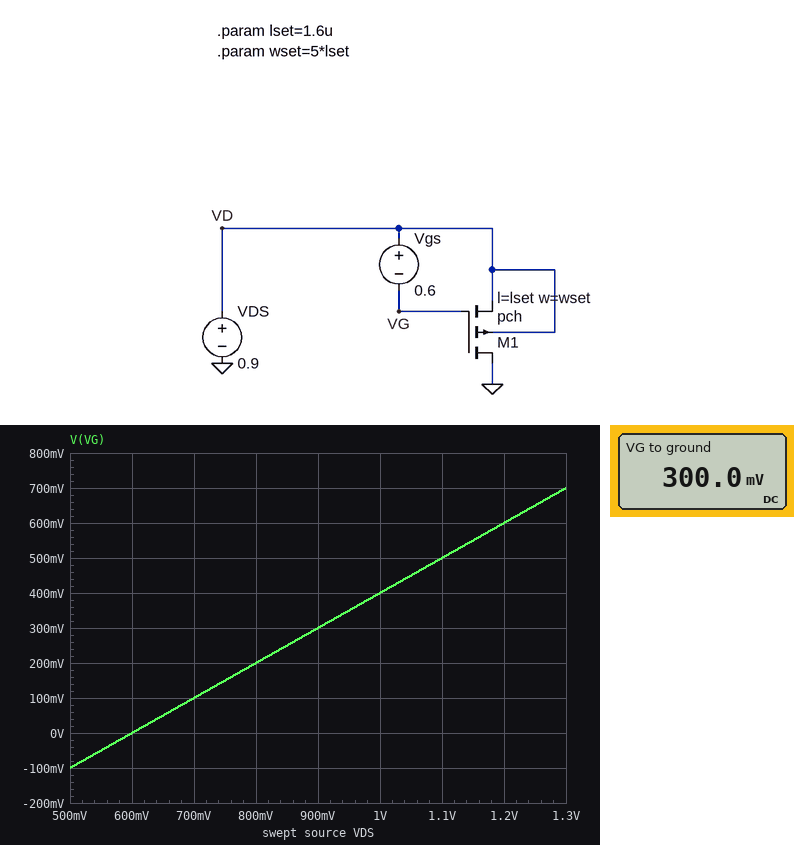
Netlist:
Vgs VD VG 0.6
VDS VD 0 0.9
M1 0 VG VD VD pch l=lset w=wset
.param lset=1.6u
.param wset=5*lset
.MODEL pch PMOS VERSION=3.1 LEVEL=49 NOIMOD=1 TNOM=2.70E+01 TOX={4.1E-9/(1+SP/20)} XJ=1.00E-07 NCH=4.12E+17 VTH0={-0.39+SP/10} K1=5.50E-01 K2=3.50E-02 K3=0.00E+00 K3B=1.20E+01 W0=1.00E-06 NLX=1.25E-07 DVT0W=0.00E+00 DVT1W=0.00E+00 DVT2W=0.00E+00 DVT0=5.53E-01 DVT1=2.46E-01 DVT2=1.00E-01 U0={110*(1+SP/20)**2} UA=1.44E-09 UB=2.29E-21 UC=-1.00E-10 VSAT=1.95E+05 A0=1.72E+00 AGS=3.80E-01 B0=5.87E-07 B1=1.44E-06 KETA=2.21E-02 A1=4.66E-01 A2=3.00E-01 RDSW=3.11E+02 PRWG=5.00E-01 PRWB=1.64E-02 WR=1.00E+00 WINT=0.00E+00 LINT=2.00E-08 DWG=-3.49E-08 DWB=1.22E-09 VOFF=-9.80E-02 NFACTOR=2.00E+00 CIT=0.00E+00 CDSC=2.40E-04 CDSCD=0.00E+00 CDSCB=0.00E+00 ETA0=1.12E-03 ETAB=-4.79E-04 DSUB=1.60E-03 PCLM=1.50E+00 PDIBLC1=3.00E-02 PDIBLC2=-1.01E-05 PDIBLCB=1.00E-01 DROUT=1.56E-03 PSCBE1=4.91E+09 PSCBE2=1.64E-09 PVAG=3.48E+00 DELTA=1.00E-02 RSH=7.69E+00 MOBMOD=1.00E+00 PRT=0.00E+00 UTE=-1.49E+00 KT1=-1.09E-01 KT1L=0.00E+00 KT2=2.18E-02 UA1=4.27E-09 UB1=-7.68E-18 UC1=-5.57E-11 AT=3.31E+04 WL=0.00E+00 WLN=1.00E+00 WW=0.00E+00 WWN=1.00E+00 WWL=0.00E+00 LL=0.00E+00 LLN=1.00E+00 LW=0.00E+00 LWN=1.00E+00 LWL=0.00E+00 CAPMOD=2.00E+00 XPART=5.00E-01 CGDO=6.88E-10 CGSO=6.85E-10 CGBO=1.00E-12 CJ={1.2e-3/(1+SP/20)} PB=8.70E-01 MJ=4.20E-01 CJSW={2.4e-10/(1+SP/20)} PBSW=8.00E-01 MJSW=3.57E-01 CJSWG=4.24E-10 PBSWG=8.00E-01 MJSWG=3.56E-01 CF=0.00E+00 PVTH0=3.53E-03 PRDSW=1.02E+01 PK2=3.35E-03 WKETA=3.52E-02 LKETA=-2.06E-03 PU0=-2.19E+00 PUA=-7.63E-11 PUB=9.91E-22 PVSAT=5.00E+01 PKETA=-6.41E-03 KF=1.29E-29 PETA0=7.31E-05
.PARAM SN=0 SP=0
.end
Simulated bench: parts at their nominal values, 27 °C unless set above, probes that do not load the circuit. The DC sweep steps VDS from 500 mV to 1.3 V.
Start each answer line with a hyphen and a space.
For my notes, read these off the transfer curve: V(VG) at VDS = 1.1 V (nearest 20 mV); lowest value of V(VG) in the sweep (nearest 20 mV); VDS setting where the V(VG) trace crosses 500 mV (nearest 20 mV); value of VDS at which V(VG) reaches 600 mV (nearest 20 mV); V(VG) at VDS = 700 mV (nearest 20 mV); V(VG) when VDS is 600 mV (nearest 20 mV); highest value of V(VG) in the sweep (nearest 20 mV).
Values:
- 500 mV
- -100 mV
- 1.10 V
- 1.20 V
- 100 mV
- 0 V
- 700 mV
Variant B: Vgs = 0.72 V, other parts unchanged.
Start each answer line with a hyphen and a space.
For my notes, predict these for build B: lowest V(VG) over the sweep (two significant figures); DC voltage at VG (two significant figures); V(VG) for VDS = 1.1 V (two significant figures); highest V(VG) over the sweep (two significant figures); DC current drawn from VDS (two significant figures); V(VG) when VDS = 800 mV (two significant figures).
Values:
- -220 mV
- 180 mV
- 380 mV
- 580 mV
- 14 µA
- 80 mV
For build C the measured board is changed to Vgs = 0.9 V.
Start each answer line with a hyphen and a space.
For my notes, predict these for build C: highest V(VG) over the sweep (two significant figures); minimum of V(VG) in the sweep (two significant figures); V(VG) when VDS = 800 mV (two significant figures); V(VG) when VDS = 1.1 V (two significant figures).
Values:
- 400 mV
- -400 mV
- -100 mV
- 200 mV
